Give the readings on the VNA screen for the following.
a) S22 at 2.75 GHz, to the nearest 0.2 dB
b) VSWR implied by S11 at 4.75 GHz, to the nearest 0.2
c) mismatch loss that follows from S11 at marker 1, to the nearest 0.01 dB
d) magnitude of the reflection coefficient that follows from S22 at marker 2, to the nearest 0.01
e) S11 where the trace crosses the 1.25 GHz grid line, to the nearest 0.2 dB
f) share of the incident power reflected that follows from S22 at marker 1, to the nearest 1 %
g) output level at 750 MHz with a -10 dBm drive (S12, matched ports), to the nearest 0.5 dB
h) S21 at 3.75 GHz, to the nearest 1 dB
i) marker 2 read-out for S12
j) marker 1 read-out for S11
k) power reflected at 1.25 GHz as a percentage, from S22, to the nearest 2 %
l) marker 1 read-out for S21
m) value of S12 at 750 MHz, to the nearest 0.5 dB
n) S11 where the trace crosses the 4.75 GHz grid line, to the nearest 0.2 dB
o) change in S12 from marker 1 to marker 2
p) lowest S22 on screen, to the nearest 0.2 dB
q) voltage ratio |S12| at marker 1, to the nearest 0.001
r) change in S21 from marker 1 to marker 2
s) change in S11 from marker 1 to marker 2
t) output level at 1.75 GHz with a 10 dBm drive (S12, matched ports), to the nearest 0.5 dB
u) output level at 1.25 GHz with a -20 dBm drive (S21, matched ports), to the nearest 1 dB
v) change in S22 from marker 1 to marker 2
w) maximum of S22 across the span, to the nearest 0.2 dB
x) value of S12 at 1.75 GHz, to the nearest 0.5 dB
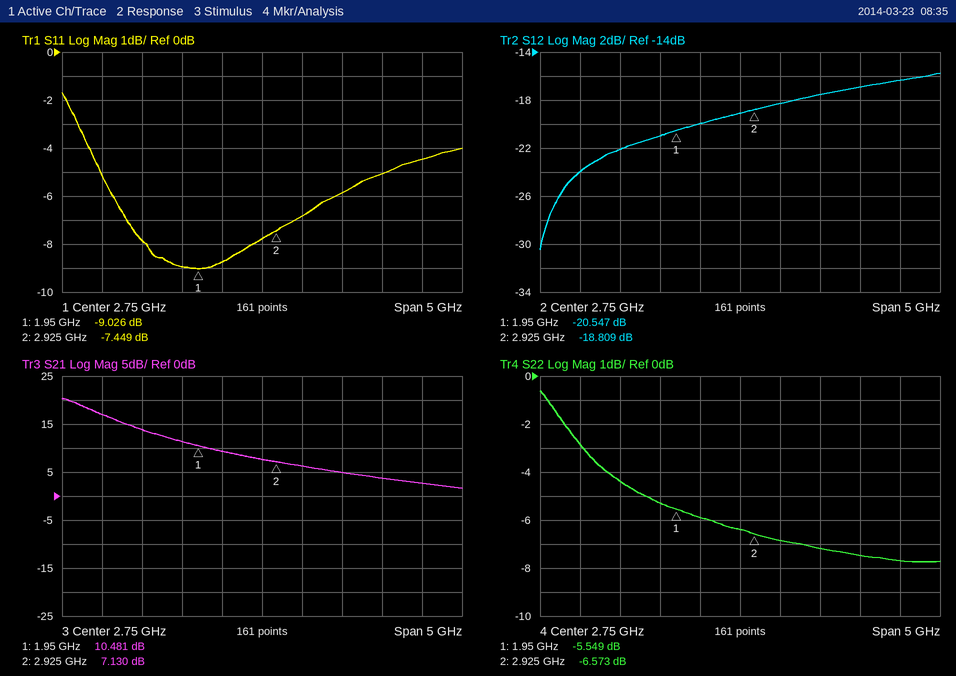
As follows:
-6.4 dB
4.0
0.58 dB
0.47
-7.8 dB
28 %
-34.0 dBm
5 dB
-18.809 dB
-9.026 dB
36 %
10.481 dB
-24.0 dB
-4.4 dB
1.738 dB
-7.8 dB
0.094
-3.351 dB
1.577 dB
-11.0 dBm
-6 dBm
-1.024 dB
-0.6 dB
-21.0 dB
